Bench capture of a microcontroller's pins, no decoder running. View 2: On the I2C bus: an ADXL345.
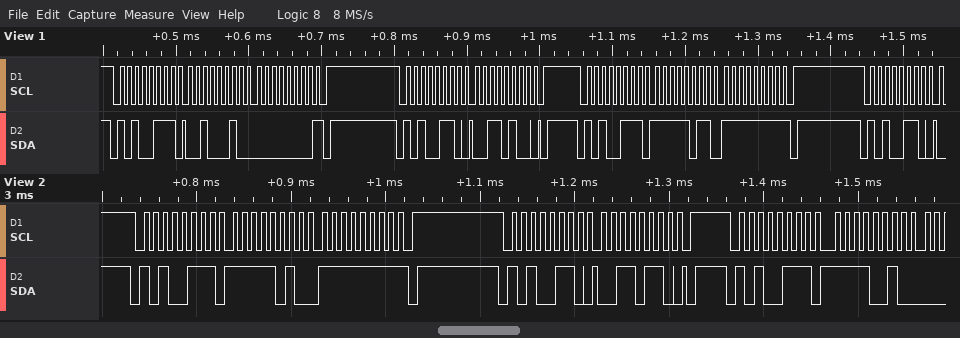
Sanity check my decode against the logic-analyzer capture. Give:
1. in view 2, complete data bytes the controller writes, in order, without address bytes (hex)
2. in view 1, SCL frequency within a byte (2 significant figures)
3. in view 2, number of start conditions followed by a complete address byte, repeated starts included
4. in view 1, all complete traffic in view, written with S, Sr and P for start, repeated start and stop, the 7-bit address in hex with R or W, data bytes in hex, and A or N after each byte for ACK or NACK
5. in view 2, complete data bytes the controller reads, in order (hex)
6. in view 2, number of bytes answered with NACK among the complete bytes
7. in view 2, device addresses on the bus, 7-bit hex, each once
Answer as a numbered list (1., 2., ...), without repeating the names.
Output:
1. 36
2. 100 kHz
3. 3
4. S 53R A 22 A 00 N P S 53W A 34 A P S 53R A FB A FF N P S 53W A
5. FA FF F2
6. 1
7. 0x53
